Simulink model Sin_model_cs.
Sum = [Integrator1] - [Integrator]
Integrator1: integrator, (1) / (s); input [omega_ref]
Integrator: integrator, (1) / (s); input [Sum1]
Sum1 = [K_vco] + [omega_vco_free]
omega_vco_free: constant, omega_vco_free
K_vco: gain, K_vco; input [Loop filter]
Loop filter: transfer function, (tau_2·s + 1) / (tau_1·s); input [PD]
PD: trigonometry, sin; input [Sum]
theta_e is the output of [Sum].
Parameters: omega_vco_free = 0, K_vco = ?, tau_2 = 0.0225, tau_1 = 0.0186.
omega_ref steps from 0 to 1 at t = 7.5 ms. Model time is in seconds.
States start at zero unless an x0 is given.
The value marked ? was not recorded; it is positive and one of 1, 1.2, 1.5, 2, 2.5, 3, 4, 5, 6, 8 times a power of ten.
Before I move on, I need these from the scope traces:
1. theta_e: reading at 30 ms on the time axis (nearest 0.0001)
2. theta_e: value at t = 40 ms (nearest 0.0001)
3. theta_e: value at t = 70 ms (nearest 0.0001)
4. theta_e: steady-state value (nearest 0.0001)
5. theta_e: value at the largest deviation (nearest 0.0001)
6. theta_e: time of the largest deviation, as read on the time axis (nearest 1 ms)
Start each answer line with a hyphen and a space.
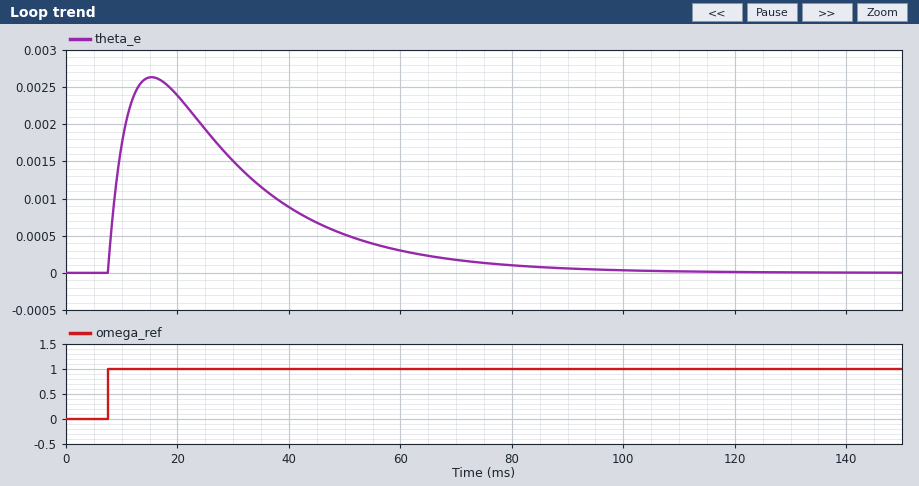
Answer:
- 0.0015
- 0.0009
- 0.0002
- 0.0000
- 0.0026
- 15 ms
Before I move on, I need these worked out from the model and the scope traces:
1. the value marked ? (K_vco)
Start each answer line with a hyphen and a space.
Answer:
- 250
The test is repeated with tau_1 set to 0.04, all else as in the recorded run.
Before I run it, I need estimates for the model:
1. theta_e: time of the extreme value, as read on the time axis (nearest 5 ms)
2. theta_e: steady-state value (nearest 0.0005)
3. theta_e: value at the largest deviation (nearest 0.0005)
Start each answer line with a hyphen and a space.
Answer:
- 20 ms
- 0.0000
- 0.0050
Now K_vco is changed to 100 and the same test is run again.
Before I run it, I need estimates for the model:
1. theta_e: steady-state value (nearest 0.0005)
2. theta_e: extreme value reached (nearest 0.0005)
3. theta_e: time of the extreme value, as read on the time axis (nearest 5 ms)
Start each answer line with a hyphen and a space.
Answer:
- 0.0000
- 0.0055
- 20 ms
